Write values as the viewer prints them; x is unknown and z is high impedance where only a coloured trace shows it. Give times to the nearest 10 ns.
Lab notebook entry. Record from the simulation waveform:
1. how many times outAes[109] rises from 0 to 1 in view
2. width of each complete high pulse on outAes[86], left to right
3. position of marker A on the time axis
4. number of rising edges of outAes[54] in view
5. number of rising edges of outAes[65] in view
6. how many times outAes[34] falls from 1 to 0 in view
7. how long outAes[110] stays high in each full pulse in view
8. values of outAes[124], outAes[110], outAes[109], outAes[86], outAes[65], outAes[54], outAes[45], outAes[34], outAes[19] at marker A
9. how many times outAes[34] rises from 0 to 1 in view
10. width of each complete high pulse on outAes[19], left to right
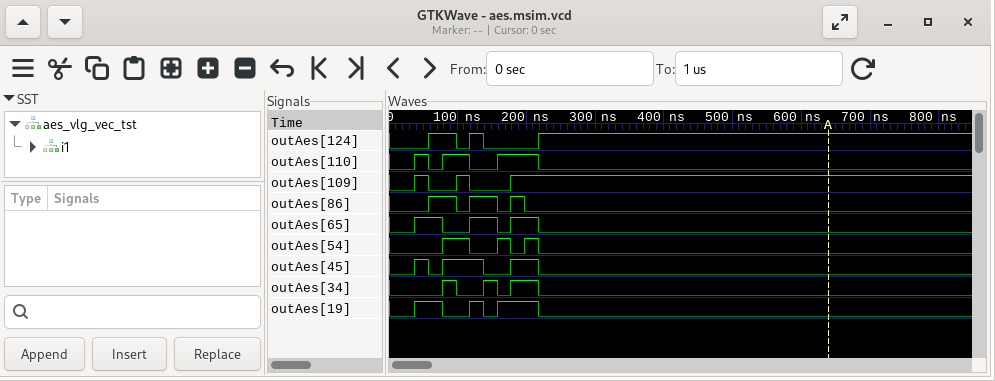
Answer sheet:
3
40 ns, 40 ns, 20 ns
640 ns
3
3
3
20 ns, 40 ns, 60 ns
outAes[124]=1, outAes[110]=0, outAes[109]=1, outAes[86]=0, outAes[65]=0, outAes[54]=0, outAes[45]=0, outAes[34]=0, outAes[19]=0
3
40 ns, 20 ns, 60 ns
